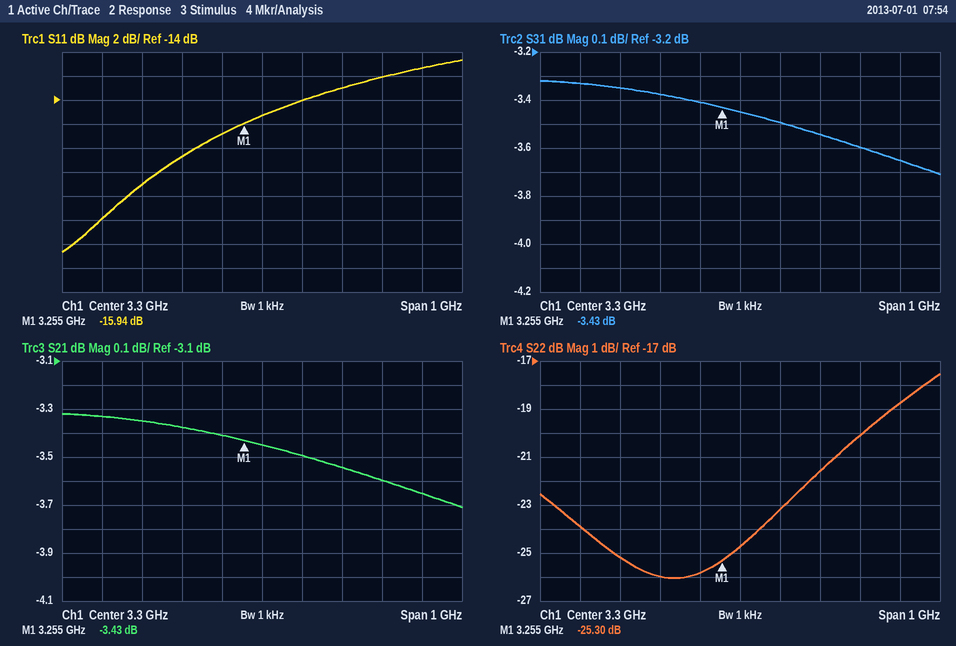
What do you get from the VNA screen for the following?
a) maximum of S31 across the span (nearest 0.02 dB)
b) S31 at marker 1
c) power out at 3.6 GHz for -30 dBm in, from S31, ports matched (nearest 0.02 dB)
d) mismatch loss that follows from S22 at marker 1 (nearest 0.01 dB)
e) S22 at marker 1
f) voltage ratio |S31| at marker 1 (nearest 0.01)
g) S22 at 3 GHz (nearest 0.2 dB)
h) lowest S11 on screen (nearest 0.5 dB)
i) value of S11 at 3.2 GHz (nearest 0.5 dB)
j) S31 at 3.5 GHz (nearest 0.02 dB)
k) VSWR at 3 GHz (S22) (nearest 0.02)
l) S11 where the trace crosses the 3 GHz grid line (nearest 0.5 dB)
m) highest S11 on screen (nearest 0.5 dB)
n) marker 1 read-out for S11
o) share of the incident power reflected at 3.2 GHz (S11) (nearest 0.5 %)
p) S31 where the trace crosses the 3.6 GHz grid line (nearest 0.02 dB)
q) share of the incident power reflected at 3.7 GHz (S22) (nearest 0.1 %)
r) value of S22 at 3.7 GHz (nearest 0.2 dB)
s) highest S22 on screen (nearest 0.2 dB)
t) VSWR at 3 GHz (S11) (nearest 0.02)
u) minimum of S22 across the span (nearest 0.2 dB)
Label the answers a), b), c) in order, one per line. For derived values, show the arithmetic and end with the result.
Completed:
a) -3.32 dB
b) -3.43 dB
c) -30 dBm + (-3.60 dB) = -33.60 dBm
d) −10 log10(1 − 10^(-25.3/10)) ≈ 0.01 dB
e) -25.30 dB
f) 10^(-3.43/20) ≈ 0.67
g) -25.2 dB
h) -26.5 dB
i) -17.0 dB
j) -3.54 dB
k) |Γ| = 10^(-25.2/20) = 0.0550; VSWR = (1 + 0.0550)/(1 − 0.0550) ≈ 1.12
l) -21.0 dB
m) -10.5 dB
n) -15.94 dB
o) 10^(-17/10) ≈ 2.0 %
p) -3.60 dB
q) 10^(-18.8/10) ≈ 1.3 %
r) -18.8 dB
s) -17.6 dB
t) |Γ| = 10^(-21/20) = 0.0891; VSWR = (1 + 0.0891)/(1 − 0.0891) ≈ 1.20
u) -26.0 dB
